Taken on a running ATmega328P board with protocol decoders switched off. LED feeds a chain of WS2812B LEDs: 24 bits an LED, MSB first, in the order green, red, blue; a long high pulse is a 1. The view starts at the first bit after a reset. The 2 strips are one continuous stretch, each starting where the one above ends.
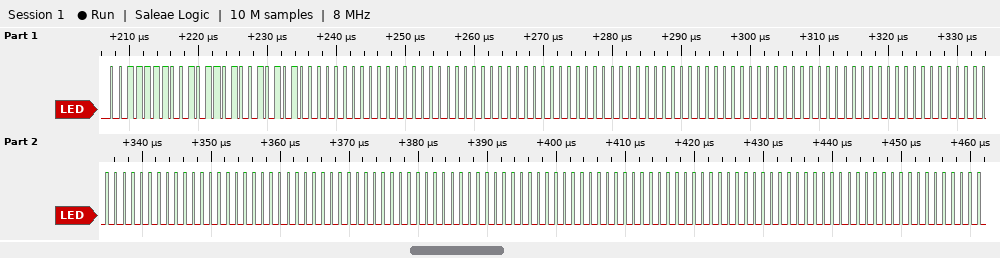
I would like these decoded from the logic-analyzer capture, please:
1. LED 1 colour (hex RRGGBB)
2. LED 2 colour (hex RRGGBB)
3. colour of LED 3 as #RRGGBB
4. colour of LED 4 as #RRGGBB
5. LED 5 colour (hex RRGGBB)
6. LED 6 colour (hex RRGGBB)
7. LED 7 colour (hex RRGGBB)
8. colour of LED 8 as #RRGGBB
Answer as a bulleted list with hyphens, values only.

- #5A3E54
- #000000
- #000000
- #000000
- #000000
- #000000
- #000000
- #000000
